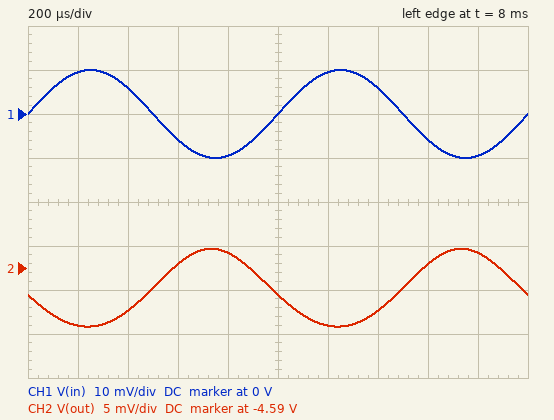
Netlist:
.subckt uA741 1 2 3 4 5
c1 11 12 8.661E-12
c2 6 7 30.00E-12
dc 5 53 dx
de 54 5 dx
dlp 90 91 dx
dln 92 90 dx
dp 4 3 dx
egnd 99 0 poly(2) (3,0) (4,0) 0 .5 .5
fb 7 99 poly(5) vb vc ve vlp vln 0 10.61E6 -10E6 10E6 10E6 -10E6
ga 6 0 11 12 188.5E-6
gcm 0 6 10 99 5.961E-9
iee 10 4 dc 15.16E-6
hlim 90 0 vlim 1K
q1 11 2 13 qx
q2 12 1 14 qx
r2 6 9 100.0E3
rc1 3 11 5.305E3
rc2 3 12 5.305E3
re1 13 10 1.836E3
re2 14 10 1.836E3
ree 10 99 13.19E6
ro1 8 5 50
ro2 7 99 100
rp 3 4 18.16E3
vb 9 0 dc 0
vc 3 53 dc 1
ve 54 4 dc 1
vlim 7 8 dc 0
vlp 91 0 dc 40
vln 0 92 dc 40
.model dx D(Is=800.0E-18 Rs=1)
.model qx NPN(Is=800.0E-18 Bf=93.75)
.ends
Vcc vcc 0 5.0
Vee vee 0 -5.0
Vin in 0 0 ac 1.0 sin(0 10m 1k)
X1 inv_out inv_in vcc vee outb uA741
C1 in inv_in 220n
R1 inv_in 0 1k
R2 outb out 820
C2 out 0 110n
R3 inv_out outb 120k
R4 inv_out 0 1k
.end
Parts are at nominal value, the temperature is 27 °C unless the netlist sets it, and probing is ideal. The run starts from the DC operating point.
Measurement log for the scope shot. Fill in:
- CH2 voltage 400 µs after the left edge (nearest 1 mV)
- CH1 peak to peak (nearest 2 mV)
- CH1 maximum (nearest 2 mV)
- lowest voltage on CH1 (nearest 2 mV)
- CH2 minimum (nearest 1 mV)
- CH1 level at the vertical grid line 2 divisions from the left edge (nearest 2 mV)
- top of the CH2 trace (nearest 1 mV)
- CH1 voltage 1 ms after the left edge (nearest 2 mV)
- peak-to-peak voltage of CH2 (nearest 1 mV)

-4.595 V
20 mV
10 mV
-10 mV
-4.597 V
6 mV
-4.588 V
0 V
9 mV
